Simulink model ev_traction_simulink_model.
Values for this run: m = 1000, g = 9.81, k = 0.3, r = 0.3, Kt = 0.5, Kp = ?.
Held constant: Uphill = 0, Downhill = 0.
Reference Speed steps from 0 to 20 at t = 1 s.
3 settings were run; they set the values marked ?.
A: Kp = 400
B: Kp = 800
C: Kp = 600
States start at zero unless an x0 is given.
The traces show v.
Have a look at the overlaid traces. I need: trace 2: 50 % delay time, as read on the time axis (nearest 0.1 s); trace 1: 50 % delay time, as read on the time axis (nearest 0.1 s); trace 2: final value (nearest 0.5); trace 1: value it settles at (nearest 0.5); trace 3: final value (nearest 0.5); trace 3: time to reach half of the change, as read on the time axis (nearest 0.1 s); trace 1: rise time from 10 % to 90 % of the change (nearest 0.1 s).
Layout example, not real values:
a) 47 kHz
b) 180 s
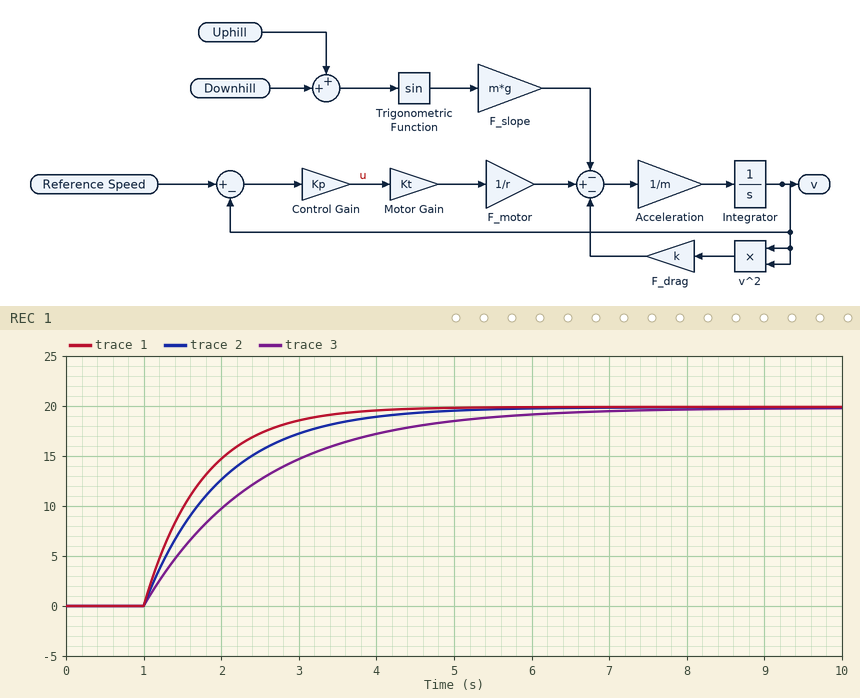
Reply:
a) 1.7 s
b) 1.5 s
c) 20.0
d) 20.0
e) 20.0
f) 2.0 s
g) 1.6 s
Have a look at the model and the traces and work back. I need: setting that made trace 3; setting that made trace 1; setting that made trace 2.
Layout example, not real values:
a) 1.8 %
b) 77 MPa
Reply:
a) A
b) B
c) C
